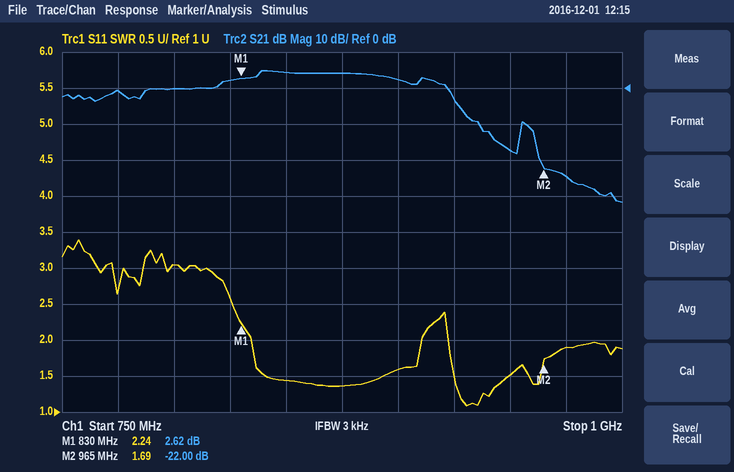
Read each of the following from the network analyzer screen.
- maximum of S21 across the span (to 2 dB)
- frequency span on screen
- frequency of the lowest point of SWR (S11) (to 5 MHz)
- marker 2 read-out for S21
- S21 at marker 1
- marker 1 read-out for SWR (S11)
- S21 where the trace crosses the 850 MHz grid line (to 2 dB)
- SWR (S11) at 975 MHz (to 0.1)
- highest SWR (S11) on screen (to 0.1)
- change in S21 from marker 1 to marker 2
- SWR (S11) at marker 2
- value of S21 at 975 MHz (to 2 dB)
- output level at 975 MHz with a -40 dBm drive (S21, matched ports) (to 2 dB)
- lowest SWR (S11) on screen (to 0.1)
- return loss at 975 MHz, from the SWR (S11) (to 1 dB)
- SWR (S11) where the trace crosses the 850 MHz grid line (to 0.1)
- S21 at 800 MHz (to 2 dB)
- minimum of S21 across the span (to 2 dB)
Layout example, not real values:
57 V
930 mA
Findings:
4 dB
250 MHz
930 MHz
-22.00 dB
2.62 dB
2.24
4 dB
1.9
3.4
-24.62 dB
1.69
-24 dB
-64 dBm
1.1
10 dB
1.4
0 dB
-32 dB
